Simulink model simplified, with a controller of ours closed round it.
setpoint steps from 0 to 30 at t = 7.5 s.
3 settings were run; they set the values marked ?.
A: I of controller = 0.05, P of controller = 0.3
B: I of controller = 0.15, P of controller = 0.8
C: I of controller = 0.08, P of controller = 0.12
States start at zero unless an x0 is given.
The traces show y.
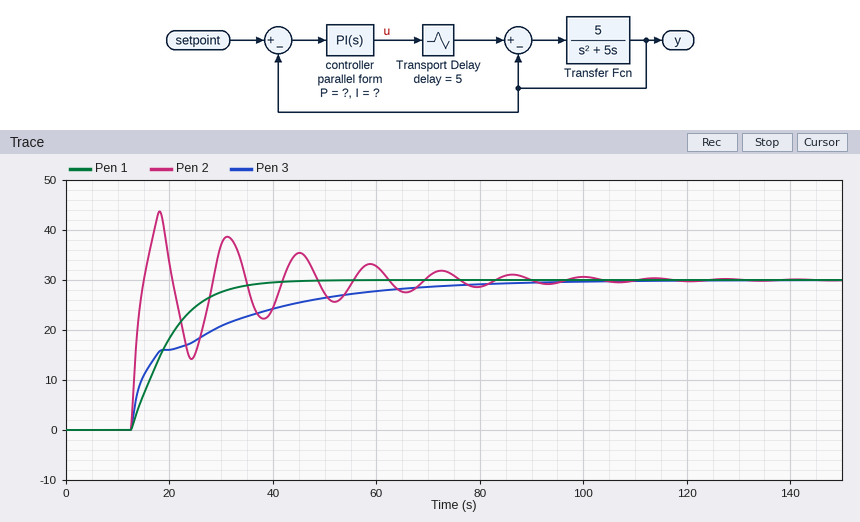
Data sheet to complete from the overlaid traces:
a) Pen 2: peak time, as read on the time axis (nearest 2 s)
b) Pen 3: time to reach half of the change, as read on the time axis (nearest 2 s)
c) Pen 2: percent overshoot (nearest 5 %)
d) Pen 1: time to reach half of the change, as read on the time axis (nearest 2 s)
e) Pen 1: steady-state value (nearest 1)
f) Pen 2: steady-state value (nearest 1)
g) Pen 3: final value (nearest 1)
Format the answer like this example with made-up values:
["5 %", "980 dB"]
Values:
["18 s", "18 s", "45 %", "18 s", "30", "30", "30"]
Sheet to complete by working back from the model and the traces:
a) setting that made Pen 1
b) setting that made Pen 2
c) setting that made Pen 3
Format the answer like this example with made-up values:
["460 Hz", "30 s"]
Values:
["C", "B", "A"]
